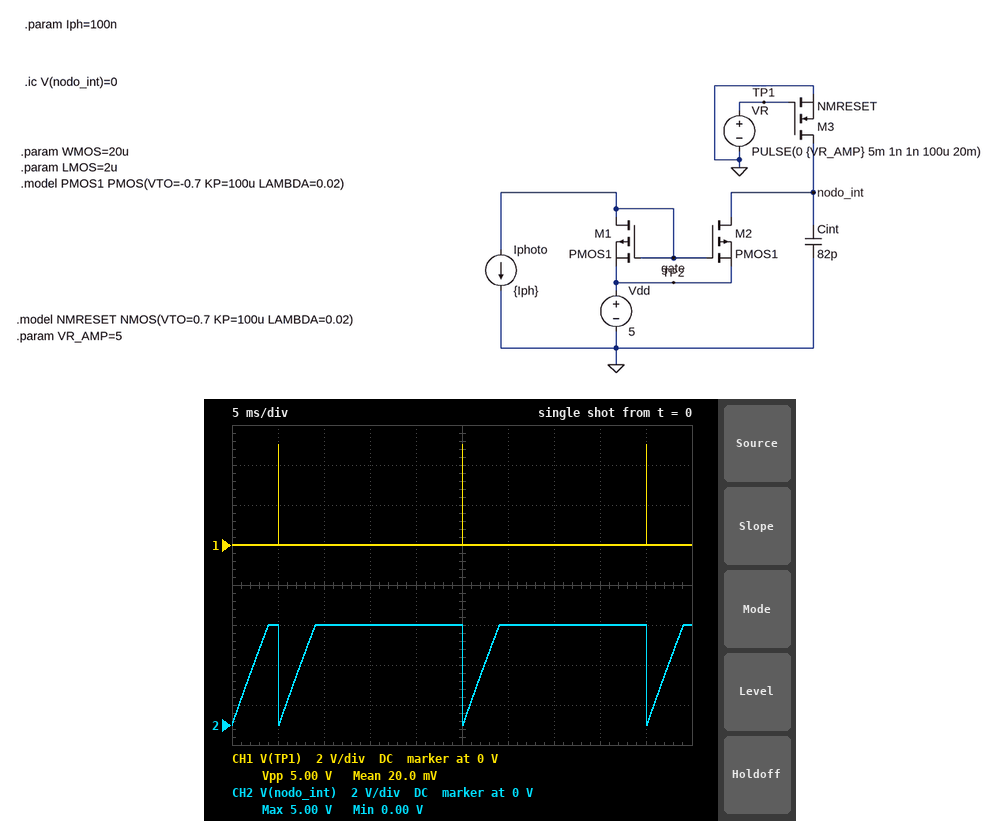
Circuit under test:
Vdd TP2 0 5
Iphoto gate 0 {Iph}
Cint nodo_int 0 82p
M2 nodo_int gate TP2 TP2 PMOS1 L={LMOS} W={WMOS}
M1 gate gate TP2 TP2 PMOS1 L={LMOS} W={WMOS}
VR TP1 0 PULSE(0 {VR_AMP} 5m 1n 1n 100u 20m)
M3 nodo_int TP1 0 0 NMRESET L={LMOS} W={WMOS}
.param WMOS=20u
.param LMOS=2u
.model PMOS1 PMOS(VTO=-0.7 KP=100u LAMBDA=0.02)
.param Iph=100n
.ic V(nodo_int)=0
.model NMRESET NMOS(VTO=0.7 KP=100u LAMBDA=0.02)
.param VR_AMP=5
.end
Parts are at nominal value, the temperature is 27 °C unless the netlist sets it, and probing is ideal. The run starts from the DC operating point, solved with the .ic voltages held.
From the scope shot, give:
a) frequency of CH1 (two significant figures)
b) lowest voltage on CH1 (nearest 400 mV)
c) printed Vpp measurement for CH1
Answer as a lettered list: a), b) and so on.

a) 50 Hz
b) 0 V
c) 5.00 V
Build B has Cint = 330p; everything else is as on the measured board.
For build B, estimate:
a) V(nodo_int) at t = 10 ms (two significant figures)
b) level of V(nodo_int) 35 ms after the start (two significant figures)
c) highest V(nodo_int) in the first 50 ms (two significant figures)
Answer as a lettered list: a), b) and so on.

a) 1.6 V
b) 3.2 V
c) 5.0 V
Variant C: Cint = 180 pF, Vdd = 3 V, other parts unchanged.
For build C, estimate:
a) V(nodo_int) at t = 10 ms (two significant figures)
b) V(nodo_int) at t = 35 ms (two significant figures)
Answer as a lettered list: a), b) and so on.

a) 2.8 V
b) 3.0 V
